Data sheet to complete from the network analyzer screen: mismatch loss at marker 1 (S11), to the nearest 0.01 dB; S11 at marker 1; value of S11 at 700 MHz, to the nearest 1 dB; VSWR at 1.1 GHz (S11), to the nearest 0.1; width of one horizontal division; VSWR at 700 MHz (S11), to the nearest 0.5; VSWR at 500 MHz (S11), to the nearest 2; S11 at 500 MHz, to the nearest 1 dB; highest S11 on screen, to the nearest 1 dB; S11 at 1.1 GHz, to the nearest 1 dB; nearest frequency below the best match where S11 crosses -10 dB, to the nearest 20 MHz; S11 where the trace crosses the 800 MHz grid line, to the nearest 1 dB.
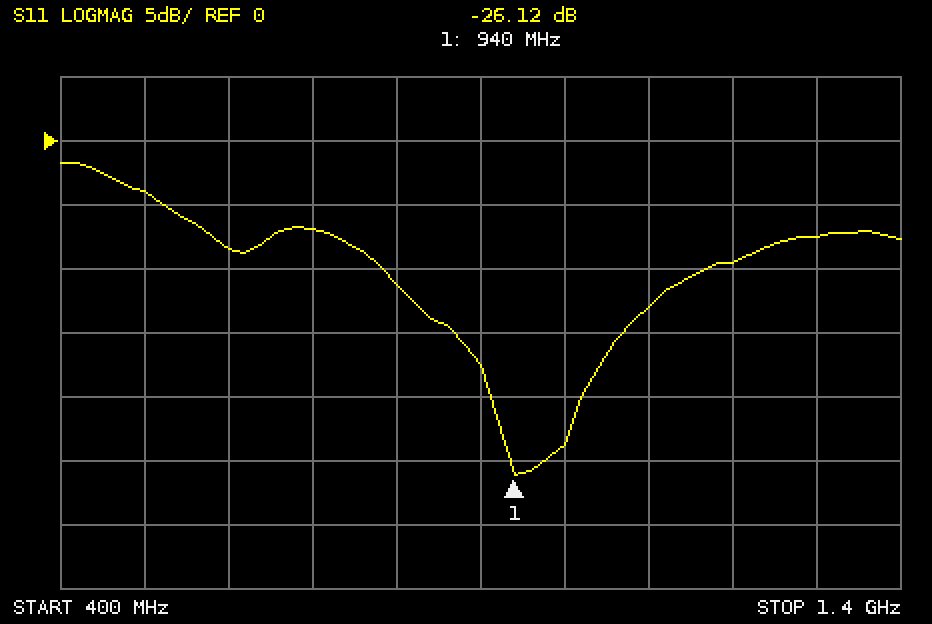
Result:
0.01 dB
-26.12 dB
-7 dB
1.6
100 MHz
2.5
4
-4 dB
-2 dB
-13 dB
780 MHz
-11 dB
